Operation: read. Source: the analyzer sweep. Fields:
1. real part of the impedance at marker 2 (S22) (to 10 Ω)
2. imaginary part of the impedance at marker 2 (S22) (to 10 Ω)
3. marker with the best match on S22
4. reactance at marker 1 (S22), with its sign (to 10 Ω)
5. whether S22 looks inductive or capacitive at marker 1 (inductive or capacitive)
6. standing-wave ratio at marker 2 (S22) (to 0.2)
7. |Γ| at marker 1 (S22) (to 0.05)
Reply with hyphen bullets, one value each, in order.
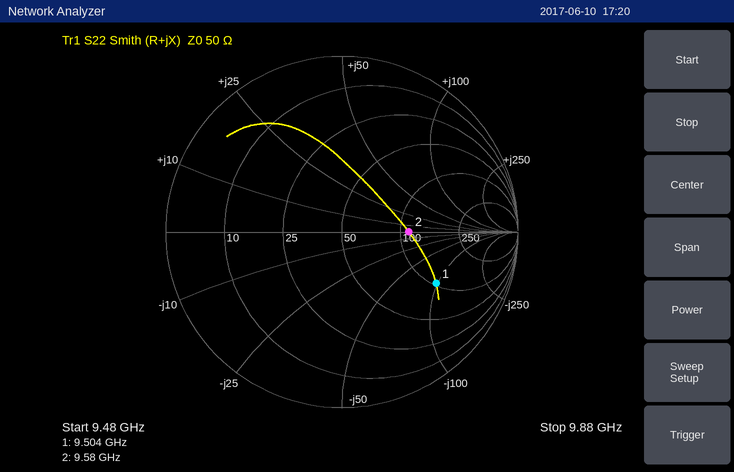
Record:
- 110 Ω
- 0 Ω
- marker 2
- -100 Ω
- capacitive
- 2.2
- 0.60
